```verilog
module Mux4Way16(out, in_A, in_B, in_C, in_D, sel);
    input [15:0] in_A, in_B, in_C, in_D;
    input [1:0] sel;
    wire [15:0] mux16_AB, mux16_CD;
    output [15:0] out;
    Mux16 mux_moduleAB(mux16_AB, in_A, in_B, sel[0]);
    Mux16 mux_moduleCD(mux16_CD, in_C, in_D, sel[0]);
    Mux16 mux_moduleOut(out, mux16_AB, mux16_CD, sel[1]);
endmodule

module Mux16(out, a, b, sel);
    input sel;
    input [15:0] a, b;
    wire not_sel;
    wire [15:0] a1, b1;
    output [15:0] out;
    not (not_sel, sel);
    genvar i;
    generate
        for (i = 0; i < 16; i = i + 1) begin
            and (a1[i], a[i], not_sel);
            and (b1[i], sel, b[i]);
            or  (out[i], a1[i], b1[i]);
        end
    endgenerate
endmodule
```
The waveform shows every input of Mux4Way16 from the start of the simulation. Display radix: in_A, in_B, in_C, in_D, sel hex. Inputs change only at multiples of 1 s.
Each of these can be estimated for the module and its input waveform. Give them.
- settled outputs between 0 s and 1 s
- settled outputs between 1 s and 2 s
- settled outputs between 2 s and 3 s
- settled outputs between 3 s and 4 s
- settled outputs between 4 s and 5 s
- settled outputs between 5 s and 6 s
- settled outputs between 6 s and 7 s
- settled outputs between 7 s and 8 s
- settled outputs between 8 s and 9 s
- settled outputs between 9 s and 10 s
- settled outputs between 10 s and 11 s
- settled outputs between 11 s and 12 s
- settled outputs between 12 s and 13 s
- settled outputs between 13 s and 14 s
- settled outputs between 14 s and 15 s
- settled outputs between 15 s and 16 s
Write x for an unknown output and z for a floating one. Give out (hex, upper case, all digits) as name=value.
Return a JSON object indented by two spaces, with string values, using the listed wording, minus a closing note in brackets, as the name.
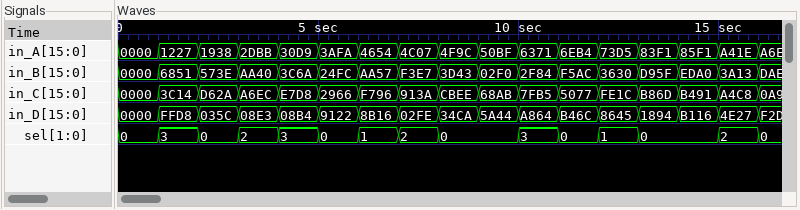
{
  "settled outputs between 0 s and 1 s": "out=0000",
  "settled outputs between 1 s and 2 s": "out=FFD8",
  "settled outputs between 2 s and 3 s": "out=1938",
  "settled outputs between 3 s and 4 s": "out=A6EC",
  "settled outputs between 4 s and 5 s": "out=08B4",
  "settled outputs between 5 s and 6 s": "out=3AFA",
  "settled outputs between 6 s and 7 s": "out=AA57",
  "settled outputs between 7 s and 8 s": "out=913A",
  "settled outputs between 8 s and 9 s": "out=4F9C",
  "settled outputs between 9 s and 10 s": "out=50BF",
  "settled outputs between 10 s and 11 s": "out=A864",
  "settled outputs between 11 s and 12 s": "out=6EB4",
  "settled outputs between 12 s and 13 s": "out=3630",
  "settled outputs between 13 s and 14 s": "out=83F1",
  "settled outputs between 14 s and 15 s": "out=85F1",
  "settled outputs between 15 s and 16 s": "out=A4C8"
}
